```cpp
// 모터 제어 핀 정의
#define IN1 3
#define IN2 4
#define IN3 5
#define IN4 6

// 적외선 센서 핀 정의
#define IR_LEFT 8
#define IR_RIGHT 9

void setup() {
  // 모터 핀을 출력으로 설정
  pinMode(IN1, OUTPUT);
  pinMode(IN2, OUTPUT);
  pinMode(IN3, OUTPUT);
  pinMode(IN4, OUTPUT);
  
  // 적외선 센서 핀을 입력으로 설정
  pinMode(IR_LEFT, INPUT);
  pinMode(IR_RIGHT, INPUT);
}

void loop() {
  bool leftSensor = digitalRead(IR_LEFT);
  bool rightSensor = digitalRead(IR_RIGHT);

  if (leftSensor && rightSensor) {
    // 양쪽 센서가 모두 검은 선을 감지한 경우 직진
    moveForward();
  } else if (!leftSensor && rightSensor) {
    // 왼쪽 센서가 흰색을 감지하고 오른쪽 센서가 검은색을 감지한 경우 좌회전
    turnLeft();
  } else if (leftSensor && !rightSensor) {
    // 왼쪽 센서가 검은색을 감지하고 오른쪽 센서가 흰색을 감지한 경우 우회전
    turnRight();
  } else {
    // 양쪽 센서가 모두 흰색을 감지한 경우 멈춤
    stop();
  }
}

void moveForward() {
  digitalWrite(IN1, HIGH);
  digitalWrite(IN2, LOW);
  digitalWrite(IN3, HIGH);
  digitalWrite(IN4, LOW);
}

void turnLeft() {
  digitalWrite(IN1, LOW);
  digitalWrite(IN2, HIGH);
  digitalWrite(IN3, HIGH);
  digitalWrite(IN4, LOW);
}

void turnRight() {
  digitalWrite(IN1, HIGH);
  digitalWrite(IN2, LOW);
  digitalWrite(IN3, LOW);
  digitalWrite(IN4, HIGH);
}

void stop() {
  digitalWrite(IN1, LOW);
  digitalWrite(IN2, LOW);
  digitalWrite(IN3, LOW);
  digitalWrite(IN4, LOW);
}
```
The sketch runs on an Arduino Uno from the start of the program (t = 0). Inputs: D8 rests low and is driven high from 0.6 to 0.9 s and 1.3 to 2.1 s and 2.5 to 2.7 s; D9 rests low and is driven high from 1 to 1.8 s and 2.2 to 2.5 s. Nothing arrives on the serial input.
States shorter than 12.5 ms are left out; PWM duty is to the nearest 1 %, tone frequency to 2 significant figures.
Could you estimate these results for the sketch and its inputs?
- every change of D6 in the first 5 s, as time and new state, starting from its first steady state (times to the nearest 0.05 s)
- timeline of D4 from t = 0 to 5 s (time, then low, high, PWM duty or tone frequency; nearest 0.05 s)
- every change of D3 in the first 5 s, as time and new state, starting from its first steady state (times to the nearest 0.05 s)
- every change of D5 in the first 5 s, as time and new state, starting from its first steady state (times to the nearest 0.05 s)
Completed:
0 s low; 0.6 s high; 0.9 s low; 1.8 s high; 2.1 s low; 2.5 s high; 2.7 s low
0 s low; 1 s high; 1.3 s low; 2.2 s high; 2.5 s low
0 s low; 0.6 s high; 0.9 s low; 1.3 s high; 2.1 s low; 2.5 s high; 2.7 s low
0 s low; 1 s high; 1.8 s low; 2.2 s high; 2.5 s low
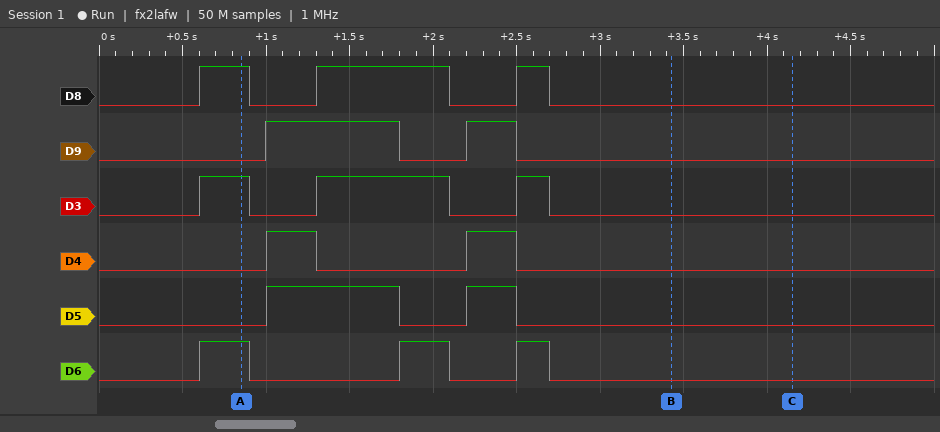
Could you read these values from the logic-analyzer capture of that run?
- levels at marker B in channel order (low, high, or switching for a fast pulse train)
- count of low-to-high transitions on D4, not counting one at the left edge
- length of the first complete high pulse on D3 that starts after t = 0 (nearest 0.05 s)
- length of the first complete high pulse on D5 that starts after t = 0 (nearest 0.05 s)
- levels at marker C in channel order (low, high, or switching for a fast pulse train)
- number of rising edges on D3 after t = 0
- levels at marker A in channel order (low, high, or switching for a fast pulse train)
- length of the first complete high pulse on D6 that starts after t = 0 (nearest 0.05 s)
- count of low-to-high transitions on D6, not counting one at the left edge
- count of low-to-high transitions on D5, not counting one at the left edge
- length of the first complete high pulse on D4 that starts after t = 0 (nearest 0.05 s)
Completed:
D8 low, D9 low, D3 low, D4 low, D5 low, D6 low
2
0.30 s
0.80 s
D8 low, D9 low, D3 low, D4 low, D5 low, D6 low
3
D8 high, D9 low, D3 high, D4 low, D5 low, D6 high
0.30 s
3
2
0.30 s
